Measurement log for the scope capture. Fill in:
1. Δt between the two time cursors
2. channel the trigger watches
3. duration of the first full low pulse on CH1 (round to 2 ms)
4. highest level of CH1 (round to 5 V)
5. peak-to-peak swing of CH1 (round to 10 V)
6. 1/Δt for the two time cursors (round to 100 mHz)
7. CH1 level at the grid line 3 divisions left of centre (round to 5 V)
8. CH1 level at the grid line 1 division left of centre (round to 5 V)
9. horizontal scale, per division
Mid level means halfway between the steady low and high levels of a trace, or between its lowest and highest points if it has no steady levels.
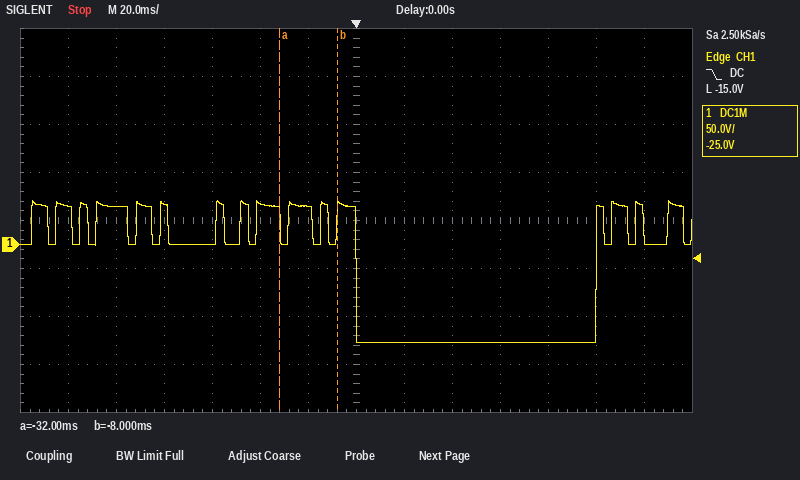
24 ms
CH1
100 ms
45 V
150 V
41.7 Hz
0 V
40 V
20 ms
